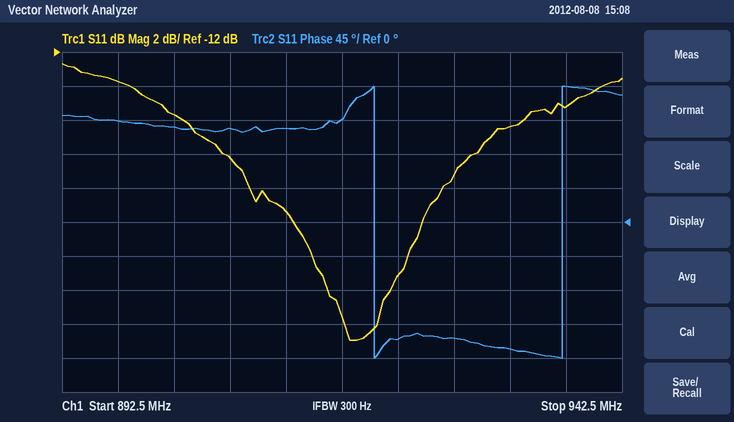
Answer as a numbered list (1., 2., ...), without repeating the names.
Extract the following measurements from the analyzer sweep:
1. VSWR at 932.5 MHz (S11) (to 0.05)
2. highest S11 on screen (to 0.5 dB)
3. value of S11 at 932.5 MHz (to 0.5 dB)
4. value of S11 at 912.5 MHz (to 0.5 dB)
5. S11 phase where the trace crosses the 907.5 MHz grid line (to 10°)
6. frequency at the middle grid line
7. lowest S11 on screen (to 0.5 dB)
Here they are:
1. 1.35
2. -12.5 dB
3. -16.5 dB
4. -21.5 dB
5. 120°
6. 917.5 MHz
7. -29.0 dB
